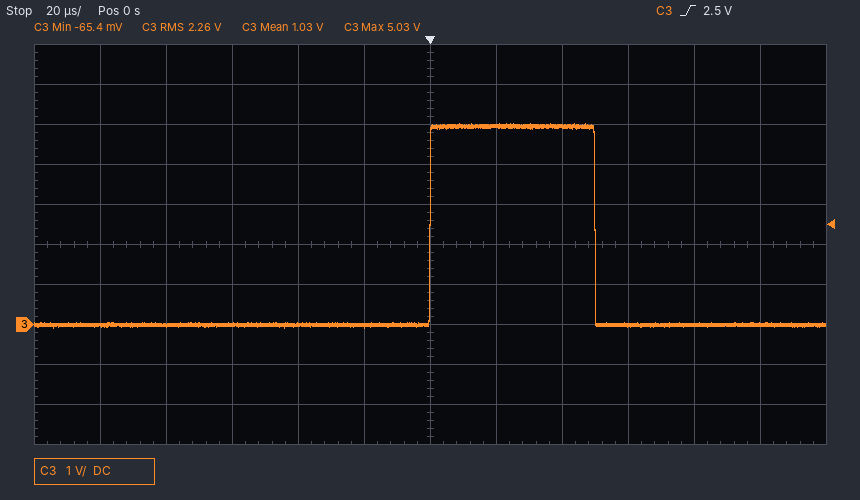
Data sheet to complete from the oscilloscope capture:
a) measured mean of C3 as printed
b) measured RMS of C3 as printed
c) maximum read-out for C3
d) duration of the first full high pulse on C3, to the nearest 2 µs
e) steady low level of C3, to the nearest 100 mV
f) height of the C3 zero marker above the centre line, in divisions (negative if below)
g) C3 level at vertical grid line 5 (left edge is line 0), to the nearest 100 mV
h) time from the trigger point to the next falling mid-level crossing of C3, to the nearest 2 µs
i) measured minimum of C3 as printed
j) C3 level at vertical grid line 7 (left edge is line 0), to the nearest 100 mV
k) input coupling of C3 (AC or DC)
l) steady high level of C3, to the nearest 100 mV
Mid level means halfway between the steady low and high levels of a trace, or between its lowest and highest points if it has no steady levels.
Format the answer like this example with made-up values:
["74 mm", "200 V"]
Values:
["1.03 V", "2.26 V", "5.03 V", "50 µs", "0.0 V", "-2.0 div", "0.0 V", "50 µs", "-65.4 mV", "5.0 V", "DC", "5.0 V"]
